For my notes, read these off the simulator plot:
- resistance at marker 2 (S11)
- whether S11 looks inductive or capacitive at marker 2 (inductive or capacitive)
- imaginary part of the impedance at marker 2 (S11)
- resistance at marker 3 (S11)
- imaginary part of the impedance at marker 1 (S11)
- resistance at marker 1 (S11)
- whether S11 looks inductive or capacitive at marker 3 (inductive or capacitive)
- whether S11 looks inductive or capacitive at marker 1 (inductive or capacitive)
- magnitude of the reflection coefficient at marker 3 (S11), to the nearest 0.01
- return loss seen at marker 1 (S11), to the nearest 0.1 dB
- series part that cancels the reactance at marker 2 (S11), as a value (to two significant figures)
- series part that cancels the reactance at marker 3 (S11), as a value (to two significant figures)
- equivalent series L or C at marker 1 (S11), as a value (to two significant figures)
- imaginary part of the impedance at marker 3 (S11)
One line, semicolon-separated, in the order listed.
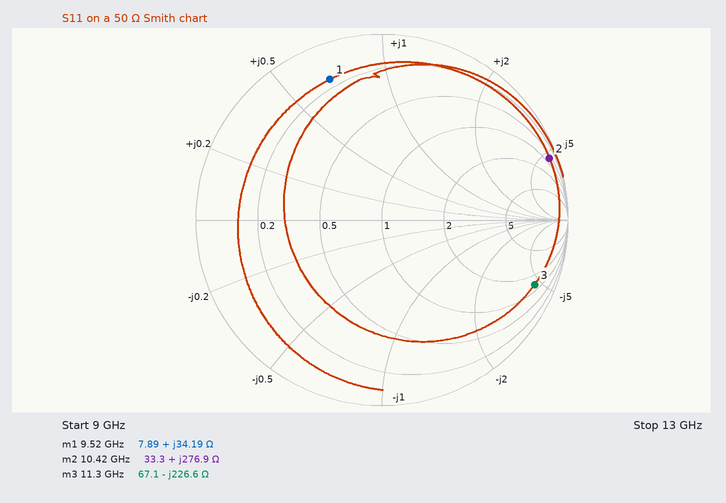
33.3 Ω; inductive; +276.9 Ω; 67.1 Ω; +34.19 Ω; 7.89 Ω; capacitive; inductive; 0.89; 1.9 dB; 55 fF; 3.2 nH; 570 pH; -226.6 Ω
